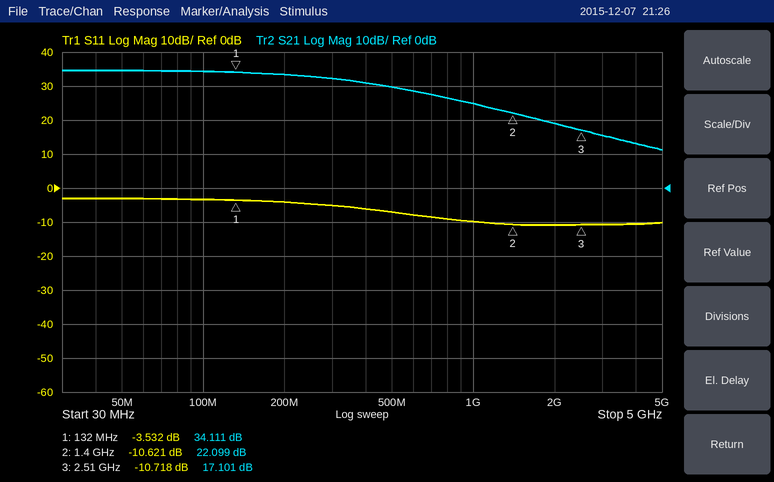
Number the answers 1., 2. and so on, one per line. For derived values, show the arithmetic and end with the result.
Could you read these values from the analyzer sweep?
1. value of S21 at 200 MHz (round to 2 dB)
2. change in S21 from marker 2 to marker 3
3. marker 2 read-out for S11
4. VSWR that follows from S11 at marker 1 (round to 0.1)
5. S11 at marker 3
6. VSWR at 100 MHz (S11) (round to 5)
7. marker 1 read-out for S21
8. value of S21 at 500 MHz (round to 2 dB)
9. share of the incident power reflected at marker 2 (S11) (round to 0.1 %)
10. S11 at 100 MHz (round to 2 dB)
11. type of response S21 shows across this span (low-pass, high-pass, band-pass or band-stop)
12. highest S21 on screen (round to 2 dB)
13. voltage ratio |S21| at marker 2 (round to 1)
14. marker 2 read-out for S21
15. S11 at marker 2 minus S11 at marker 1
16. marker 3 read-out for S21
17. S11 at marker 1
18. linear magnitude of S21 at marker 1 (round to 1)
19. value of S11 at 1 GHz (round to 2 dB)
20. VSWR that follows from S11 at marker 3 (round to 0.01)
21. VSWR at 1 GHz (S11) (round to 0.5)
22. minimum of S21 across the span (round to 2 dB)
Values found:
1. 34 dB
2. 17.101 − (22.099) = -4.998 dB
3. -10.621 dB
4. (1 + 0.6659)/(1 − 0.6659) ≈ 5.0
5. -10.718 dB
6. |Γ| = 10^(-4/20) = 0.6310; VSWR = (1 + 0.6310)/(1 − 0.6310) ≈ 4.42, so 5 to the nearest 5
7. 34.111 dB
8. 30 dB
9. 10^(-10.621/10) ≈ 8.7 %
10. -4 dB
11. low-pass
12. 34 dB
13. 10^(22.099/20) ≈ 13
14. 22.099 dB
15. -10.621 − (-3.532) = -7.089 dB
16. 17.101 dB
17. -3.532 dB
18. 10^(34.111/20) ≈ 51
19. -10 dB
20. (1 + 0.2911)/(1 − 0.2911) ≈ 1.82
21. |Γ| = 10^(-10/20) = 0.3162; VSWR = (1 + 0.3162)/(1 − 0.3162) ≈ 1.92, so 2.0 to the nearest 0.5
22. 12 dB
